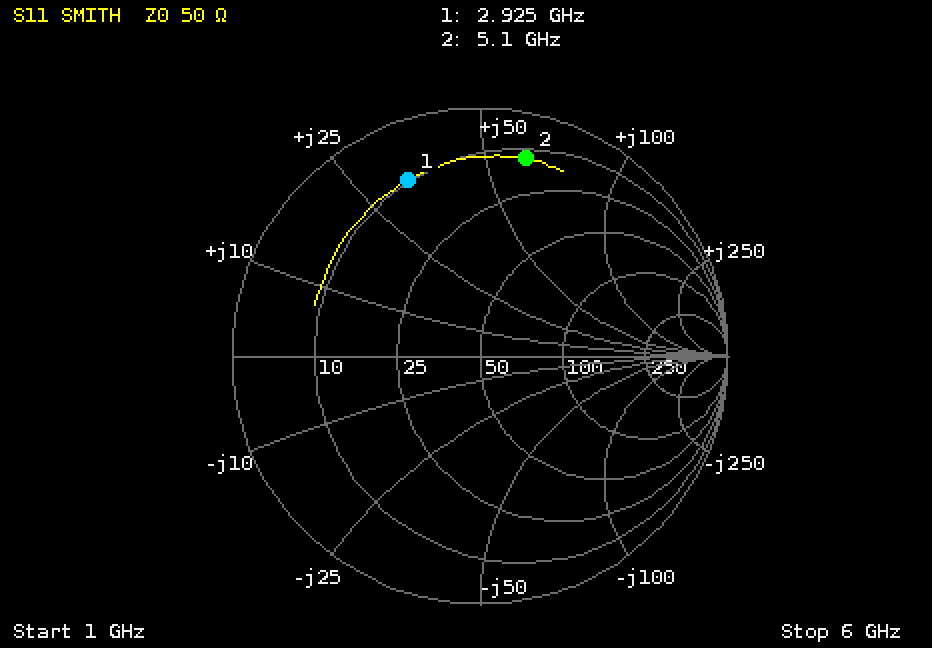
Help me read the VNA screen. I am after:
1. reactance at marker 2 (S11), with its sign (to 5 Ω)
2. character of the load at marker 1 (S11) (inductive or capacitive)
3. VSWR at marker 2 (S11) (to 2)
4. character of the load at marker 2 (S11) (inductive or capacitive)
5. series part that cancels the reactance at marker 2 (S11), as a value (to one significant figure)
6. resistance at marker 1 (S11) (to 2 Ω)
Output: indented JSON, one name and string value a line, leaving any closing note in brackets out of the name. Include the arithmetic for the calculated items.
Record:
{
  "reactance at marker 2 (S11), with its sign": "+60 Ω",
  "character of the load at marker 1 (S11)": "inductive",
  "VSWR at marker 2 (S11)": "10",
  "character of the load at marker 2 (S11)": "inductive",
  "series part that cancels the reactance at marker 2 (S11), as a value": "C = 1/(2π × 5.1 GHz × 60 Ω) ≈ 520 fF, so 500 fF to one significant figure",
  "resistance at marker 1 (S11)": "10 Ω"
}
